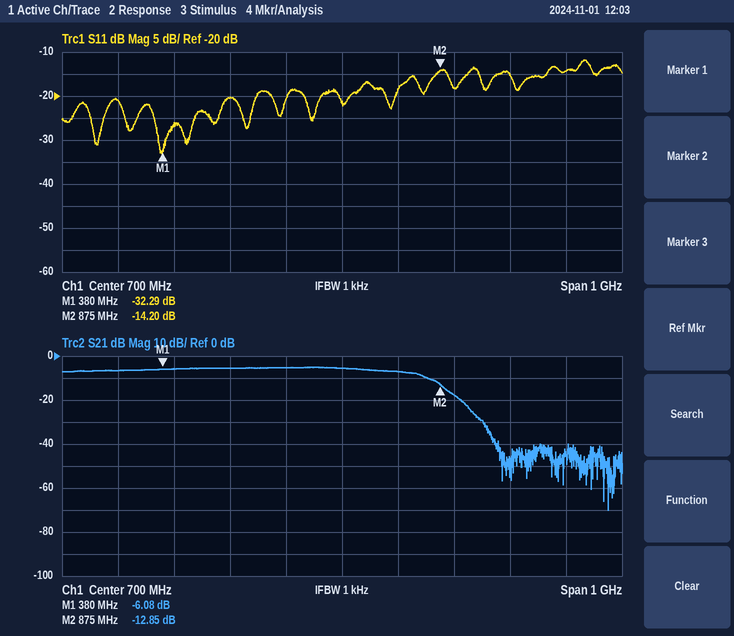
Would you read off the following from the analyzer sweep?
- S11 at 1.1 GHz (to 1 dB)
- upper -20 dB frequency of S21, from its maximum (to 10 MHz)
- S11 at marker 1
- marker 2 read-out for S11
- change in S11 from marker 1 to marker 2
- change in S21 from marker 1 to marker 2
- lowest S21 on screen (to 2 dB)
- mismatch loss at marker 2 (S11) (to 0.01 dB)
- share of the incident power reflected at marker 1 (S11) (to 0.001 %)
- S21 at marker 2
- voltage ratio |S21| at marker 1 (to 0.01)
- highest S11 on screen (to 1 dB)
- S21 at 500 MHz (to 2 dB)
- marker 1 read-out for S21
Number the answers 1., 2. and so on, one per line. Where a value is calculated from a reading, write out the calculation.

1. -14 dB
2. 930 MHz
3. -32.29 dB
4. -14.20 dB
5. -14.2 − (-32.29) = 18.09 dB
6. -12.85 − (-6.08) = -6.77 dB
7. -70 dB
8. −10 log10(1 − 10^(-14.2/10)) ≈ 0.17 dB
9. 10^(-32.29/10) ≈ 0.059 %
10. -12.85 dB
11. 10^(-6.08/20) ≈ 0.50
12. -12 dB
13. -6 dB
14. -6.08 dB
